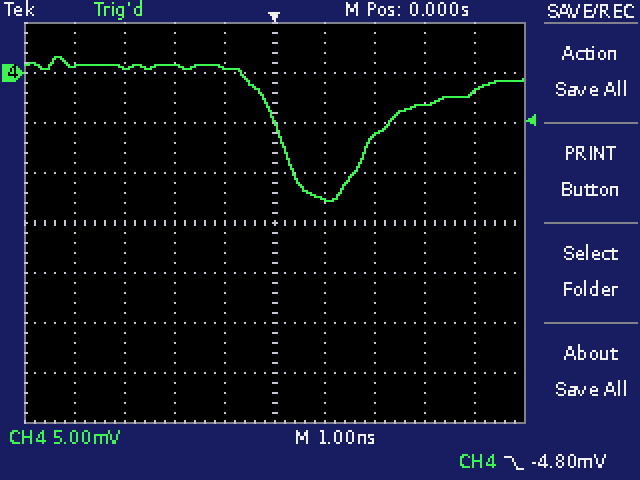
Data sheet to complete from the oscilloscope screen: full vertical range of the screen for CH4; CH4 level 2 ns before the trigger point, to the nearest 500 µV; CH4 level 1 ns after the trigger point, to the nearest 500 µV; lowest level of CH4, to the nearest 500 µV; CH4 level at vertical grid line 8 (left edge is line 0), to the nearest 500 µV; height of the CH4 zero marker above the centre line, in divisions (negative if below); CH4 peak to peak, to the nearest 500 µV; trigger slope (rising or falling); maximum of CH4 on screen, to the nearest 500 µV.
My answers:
40 mV
1.0 mV
-12.5 mV
-13.0 mV
-3.0 mV
+3.0 div
14.5 mV
falling
1.5 mV
